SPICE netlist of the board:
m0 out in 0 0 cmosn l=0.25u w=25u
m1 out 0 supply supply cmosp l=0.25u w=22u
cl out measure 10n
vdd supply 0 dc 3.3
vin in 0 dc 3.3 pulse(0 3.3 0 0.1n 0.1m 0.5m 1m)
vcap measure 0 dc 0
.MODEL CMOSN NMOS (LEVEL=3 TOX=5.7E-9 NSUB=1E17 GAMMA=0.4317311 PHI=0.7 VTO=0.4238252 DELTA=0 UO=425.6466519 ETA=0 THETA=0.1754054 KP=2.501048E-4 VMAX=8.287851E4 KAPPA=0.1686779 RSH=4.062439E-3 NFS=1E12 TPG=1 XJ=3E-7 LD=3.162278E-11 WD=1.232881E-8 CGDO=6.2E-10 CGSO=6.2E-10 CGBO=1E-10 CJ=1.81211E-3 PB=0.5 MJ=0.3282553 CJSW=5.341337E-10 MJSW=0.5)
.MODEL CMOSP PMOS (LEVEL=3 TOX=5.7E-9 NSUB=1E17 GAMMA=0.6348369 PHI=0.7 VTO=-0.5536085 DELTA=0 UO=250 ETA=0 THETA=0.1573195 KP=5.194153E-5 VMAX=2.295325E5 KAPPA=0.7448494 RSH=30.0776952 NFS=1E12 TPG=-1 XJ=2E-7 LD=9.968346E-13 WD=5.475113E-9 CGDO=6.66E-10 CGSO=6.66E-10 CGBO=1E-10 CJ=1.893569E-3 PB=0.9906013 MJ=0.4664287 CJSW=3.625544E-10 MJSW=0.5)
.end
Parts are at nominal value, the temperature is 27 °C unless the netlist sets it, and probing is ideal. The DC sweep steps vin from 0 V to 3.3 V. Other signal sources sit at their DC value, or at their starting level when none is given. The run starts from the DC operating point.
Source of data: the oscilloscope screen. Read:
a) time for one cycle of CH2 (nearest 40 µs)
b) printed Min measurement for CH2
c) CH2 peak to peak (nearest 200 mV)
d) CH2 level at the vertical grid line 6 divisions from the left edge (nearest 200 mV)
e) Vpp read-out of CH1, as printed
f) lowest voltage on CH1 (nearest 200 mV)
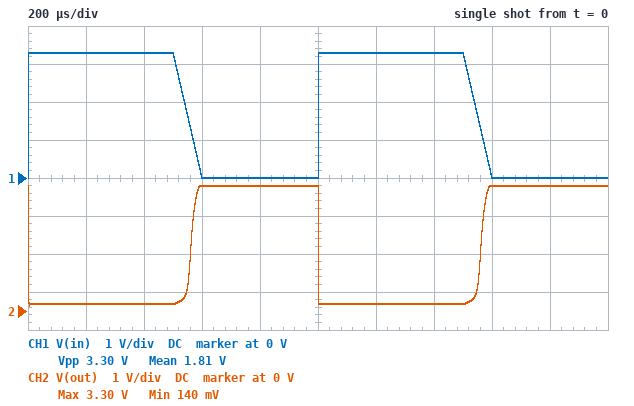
1.00 ms
140 mV
3.2 V
200 mV
3.30 V
0 V
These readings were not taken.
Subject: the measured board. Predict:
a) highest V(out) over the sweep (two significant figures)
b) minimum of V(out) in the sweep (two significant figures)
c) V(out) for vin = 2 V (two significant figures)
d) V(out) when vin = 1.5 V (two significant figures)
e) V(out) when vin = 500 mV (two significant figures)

3.3 V
180 mV
380 mV
1.5 V
3.2 V
